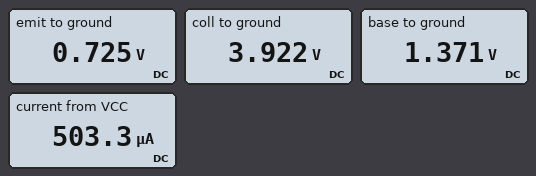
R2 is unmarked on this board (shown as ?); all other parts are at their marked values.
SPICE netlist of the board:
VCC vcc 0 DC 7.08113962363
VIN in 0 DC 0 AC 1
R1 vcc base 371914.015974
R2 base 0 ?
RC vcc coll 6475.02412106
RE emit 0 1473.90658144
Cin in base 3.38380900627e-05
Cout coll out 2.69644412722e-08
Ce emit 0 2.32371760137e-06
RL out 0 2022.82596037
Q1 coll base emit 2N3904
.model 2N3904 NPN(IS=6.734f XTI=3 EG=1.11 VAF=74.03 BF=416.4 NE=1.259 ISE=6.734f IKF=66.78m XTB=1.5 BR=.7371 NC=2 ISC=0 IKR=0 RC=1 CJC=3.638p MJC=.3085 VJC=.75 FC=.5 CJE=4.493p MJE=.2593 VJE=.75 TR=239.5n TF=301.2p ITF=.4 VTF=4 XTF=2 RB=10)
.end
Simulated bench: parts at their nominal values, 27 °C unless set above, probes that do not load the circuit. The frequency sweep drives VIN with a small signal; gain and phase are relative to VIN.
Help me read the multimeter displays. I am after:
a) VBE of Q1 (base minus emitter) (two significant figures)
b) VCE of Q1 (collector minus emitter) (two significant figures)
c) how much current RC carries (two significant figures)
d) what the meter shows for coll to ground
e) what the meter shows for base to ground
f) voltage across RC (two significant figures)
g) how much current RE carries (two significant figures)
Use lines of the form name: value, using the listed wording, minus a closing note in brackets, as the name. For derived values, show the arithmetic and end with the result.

VBE of Q1 (base minus emitter): 1.371 V - 725 mV = 650 mV
VCE of Q1 (collector minus emitter): 3.922 V - 725 mV = 3.2 V
how much current RC carries: (7.081 V - 3.922 V) / 6.475 kΩ = 490 µA
what the meter shows for coll to ground: 3.922 V
what the meter shows for base to ground: 1.371 V
voltage across RC: 7.081 V - 3.922 V = 3.2 V
how much current RE carries: (725 mV) / 1.474 kΩ = 490 µA
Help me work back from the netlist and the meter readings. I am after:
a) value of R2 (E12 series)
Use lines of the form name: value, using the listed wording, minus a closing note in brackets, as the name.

value of R2: 120 kΩ
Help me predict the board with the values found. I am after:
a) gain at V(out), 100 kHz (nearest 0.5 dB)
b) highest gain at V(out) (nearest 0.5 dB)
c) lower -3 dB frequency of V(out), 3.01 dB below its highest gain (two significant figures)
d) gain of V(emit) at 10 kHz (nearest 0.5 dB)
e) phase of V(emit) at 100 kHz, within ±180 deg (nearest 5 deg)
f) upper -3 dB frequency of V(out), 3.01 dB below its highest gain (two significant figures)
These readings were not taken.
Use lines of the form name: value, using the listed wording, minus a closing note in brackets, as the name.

gain at V(out), 100 kHz: 29.0 dB
highest gain at V(out): 29.0 dB
lower -3 dB frequency of V(out), 3.01 dB below its highest gain: 1.6 kHz
gain of V(emit) at 10 kHz: -18.0 dB
phase of V(emit) at 100 kHz, within ±180 deg: -90 deg
upper -3 dB frequency of V(out), 3.01 dB below its highest gain: 38 MHz
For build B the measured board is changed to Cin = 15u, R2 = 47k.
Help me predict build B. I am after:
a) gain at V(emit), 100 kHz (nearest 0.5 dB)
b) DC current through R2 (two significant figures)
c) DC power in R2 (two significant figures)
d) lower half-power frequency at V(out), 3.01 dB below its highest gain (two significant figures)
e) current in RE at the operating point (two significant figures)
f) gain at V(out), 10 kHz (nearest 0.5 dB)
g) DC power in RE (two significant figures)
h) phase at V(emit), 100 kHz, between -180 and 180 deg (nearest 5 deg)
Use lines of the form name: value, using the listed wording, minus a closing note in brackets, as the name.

gain at V(emit), 100 kHz: -51.5 dB
DC current through R2: 16 µA
DC power in R2: 12 µW
lower half-power frequency at V(out), 3.01 dB below its highest gain: 810 Hz
current in RE at the operating point: 100 µA
gain at V(out), 10 kHz: 15.5 dB
DC power in RE: 15 µW
phase at V(emit), 100 kHz, between -180 and 180 deg: -90 deg
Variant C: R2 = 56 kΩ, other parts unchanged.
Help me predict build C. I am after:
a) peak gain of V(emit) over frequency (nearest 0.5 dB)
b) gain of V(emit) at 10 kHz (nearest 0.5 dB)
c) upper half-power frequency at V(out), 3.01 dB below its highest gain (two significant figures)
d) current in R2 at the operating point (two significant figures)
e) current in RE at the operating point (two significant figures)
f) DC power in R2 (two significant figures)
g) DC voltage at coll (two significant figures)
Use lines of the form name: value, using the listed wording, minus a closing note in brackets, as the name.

peak gain of V(emit) over frequency: -1.0 dB
gain of V(emit) at 10 kHz: -27.5 dB
upper half-power frequency at V(out), 3.01 dB below its highest gain: 51 MHz
current in R2 at the operating point: 15 µA
current in RE at the operating point: 160 µA
DC power in R2: 13 µW
DC voltage at coll: 6.0 V
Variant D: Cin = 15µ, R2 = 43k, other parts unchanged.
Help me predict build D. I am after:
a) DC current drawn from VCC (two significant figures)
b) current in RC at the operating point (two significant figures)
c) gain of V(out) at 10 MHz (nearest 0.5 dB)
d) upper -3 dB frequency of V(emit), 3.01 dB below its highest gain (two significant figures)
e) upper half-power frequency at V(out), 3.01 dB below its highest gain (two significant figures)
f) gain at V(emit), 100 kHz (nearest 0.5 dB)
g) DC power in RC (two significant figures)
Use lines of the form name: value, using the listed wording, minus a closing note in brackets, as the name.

DC current drawn from VCC: 90 µA
current in RC at the operating point: 73 µA
gain of V(out) at 10 MHz: 12.5 dB
upper -3 dB frequency of V(emit), 3.01 dB below its highest gain: 240 Hz
upper half-power frequency at V(out), 3.01 dB below its highest gain: 57 MHz
gain at V(emit), 100 kHz: -54.0 dB
DC power in RC: 35 µW
